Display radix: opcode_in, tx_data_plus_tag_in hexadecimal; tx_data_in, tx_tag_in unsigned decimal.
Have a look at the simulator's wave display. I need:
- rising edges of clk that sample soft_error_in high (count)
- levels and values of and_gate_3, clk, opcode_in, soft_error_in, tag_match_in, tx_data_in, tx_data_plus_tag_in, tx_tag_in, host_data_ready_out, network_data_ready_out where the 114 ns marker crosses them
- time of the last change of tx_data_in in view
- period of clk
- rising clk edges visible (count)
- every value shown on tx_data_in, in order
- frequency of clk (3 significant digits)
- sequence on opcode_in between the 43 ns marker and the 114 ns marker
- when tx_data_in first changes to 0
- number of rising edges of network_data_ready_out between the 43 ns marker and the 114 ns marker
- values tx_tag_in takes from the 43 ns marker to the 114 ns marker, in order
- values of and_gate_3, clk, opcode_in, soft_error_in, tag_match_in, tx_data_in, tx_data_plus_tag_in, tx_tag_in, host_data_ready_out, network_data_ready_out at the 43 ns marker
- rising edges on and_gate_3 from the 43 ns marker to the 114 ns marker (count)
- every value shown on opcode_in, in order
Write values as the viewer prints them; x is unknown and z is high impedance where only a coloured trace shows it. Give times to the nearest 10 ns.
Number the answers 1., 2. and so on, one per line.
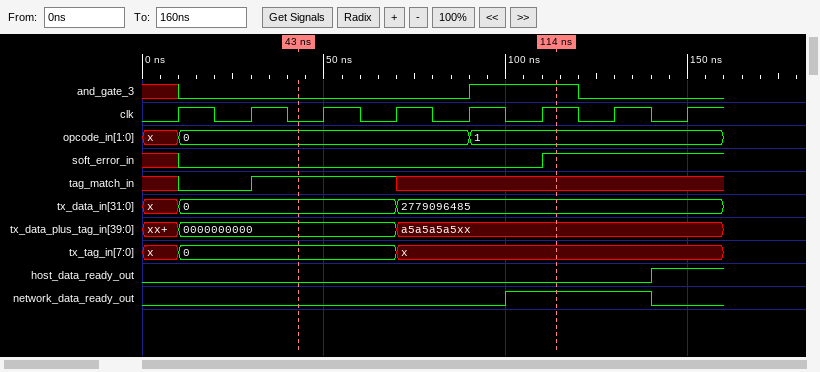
1. 2
2. and_gate_3=1, clk=1, opcode_in=1, soft_error_in=1, tag_match_in=x, tx_data_in=2779096485, tx_data_plus_tag_in=a5a5a5a5xx, tx_tag_in=x, host_data_ready_out=0, network_data_ready_out=1
3. 70 ns
4. 20 ns
5. 8
6. x, 0, 2779096485
7. 50.0 MHz
8. 0, 1
9. 10 ns
10. 1
11. 0, x
12. and_gate_3=0, clk=0, opcode_in=0, soft_error_in=0, tag_match_in=1, tx_data_in=0, tx_data_plus_tag_in=0000000000, tx_tag_in=0, host_data_ready_out=0, network_data_ready_out=0
13. 1
14. x, 0, 1
